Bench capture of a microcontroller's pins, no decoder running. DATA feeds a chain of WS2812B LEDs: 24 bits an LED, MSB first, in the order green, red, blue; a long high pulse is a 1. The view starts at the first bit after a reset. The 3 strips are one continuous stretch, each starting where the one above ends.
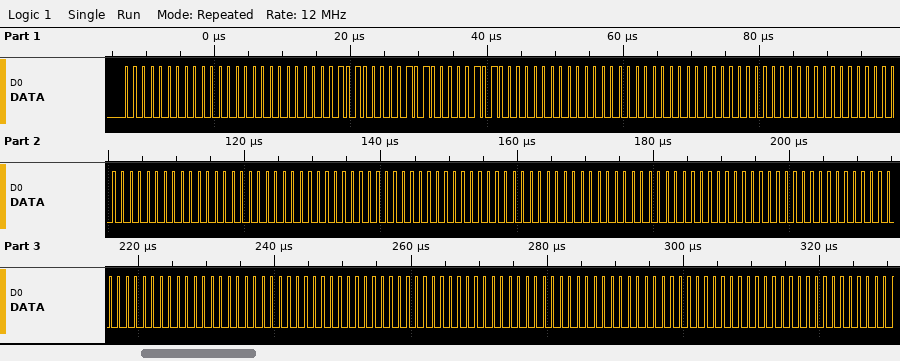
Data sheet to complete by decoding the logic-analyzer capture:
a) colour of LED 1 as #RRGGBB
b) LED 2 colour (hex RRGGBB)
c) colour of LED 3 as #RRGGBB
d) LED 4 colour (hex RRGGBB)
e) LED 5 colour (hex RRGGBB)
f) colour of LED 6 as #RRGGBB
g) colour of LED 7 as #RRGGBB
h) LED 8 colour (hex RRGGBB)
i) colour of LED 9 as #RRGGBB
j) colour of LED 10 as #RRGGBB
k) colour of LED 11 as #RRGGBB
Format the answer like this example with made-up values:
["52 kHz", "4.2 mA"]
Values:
["#000000", "#505050", "#000000", "#000000", "#000000", "#000000", "#000000", "#000000", "#000000", "#000000", "#000000"]
